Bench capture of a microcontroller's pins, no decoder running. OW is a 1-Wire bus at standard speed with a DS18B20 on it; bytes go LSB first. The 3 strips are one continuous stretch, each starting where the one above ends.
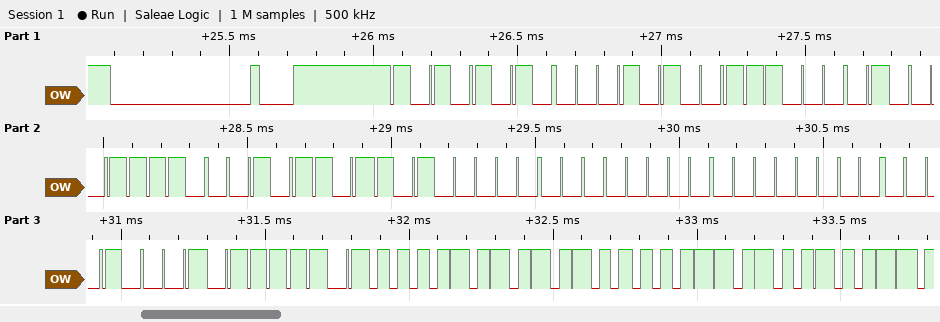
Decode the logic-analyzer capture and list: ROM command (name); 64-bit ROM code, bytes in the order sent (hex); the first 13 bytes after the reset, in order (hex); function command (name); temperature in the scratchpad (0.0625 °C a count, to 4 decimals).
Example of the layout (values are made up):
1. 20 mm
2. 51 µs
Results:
1. Match ROM
2. 28 87 78 B4 05 00 00 88
3. 55 28 87 78 B4 05 00 00 88 BE 50 05 4B
4. Read Scratchpad
5. 85.0000 °C
